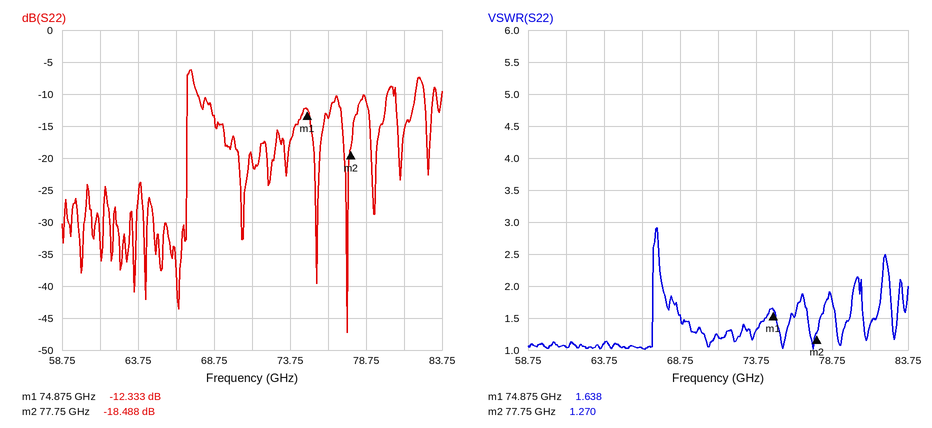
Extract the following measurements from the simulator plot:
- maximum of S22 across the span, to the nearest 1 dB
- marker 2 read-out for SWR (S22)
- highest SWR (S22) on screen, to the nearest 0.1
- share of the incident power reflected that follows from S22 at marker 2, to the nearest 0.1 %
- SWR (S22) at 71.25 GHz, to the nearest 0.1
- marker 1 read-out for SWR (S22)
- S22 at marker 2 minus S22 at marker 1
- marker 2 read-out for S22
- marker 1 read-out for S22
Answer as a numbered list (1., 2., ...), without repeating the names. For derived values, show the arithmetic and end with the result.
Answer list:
1. -6 dB
2. 1.270
3. 2.9
4. 10^(-18.488/10) ≈ 1.4 %
5. 1.2
6. 1.638
7. -18.488 − (-12.333) = -6.155 dB
8. -18.488 dB
9. -12.333 dB
